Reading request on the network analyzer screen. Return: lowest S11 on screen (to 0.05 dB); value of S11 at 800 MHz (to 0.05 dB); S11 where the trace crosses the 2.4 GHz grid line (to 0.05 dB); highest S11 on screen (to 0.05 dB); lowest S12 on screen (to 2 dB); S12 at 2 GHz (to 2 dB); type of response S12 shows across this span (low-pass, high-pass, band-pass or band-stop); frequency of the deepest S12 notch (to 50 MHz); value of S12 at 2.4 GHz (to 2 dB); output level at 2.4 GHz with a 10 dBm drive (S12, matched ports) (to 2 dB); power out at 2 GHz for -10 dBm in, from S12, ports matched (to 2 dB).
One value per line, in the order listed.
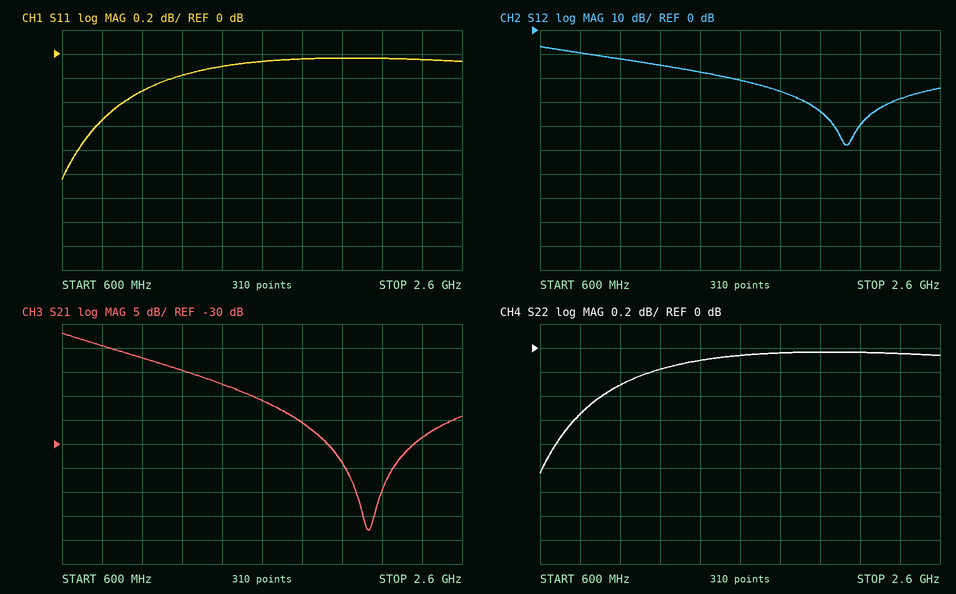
-1.05 dB
-0.55 dB
-0.05 dB
-0.05 dB
-48 dB
-34 dB
low-pass
2.15 GHz
-28 dB
-18 dBm
-44 dBm
